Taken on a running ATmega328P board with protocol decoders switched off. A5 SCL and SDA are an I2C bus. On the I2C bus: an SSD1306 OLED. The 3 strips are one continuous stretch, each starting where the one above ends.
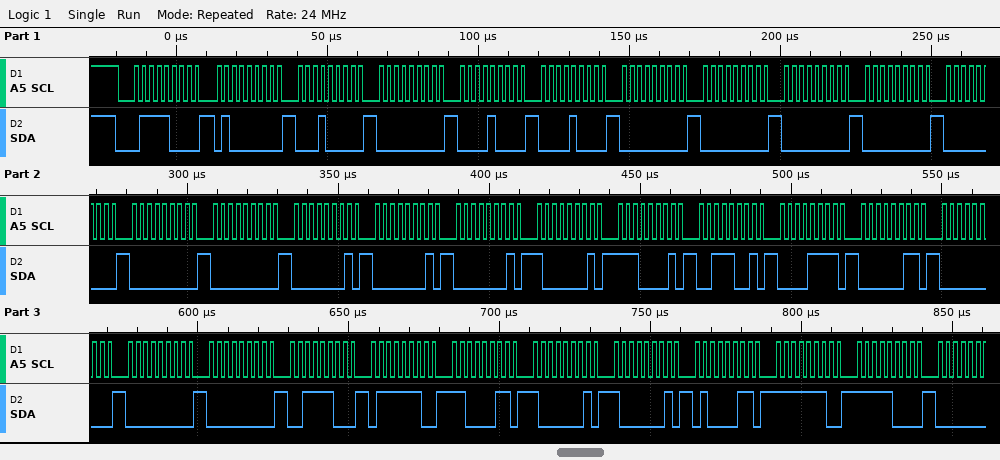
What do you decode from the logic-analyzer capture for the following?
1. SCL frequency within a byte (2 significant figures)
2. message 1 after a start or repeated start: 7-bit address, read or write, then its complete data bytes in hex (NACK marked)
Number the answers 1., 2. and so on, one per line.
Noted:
1. 400 kHz
2. 0x3C write: 40 10 00 08 08 00 00 00 00 00 00 00 01 01 01 81 E1 39 0F 03 00 00 00 3C 7E C3 81 81 43 FE F8
